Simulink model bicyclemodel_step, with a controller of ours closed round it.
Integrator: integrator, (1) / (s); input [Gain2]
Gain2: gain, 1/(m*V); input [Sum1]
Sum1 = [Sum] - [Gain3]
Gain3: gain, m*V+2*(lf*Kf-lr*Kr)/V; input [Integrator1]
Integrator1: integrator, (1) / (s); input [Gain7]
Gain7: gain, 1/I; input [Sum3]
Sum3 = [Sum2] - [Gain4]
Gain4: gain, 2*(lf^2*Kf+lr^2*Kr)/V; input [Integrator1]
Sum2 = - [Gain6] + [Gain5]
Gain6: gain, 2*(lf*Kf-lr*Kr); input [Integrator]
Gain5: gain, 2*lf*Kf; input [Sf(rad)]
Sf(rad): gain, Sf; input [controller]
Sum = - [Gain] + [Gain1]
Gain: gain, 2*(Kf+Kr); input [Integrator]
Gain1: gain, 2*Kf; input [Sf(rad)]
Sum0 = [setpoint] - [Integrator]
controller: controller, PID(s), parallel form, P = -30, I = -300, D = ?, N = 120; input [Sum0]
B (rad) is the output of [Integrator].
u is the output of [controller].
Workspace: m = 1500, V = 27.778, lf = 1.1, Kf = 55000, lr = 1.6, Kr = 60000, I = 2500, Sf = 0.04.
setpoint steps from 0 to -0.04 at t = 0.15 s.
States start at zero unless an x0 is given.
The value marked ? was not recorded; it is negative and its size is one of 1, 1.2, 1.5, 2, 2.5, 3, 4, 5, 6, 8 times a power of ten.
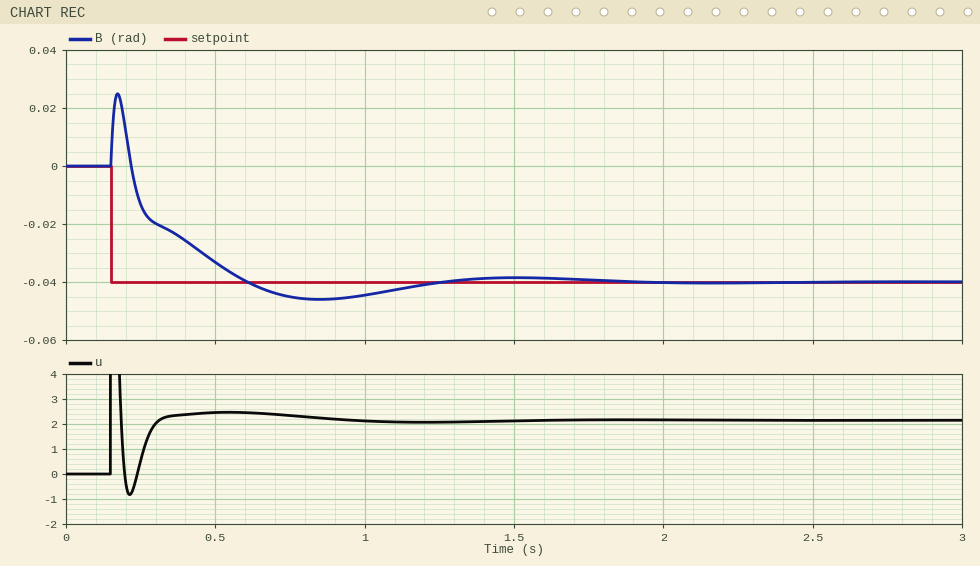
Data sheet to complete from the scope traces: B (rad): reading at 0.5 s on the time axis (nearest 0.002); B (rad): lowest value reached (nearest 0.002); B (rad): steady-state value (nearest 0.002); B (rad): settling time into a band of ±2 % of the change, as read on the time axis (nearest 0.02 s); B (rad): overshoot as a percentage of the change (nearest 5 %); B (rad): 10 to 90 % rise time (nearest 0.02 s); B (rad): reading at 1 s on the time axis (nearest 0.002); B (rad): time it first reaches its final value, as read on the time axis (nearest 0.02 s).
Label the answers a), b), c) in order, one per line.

a) -0.034
b) -0.046
c) -0.040
d) 1.74 s
e) 15 %
f) 0.32 s
g) -0.044
h) 0.60 s
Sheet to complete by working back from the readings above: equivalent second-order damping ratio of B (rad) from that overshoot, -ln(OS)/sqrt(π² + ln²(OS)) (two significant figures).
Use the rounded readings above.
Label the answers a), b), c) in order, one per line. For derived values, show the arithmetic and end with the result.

a) ln(0.15) = -1.897; 1.897 / sqrt(9.870 + 3.599) = 0.52
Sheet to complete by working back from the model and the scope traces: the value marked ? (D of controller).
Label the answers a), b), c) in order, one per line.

a) -5
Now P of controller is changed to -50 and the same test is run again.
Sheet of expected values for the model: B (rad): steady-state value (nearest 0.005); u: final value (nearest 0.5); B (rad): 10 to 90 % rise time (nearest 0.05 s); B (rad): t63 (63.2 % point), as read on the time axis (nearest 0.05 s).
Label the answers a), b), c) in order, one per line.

a) -0.040
b) 2.0
c) 0.25 s
d) 0.30 s
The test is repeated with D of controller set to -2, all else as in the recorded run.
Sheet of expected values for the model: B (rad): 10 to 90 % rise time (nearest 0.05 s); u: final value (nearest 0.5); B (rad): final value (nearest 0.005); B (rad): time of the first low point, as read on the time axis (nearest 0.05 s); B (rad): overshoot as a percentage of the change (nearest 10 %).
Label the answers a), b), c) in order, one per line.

a) 0.20 s
b) 2.0
c) -0.040
d) 0.70 s
e) 30 %
